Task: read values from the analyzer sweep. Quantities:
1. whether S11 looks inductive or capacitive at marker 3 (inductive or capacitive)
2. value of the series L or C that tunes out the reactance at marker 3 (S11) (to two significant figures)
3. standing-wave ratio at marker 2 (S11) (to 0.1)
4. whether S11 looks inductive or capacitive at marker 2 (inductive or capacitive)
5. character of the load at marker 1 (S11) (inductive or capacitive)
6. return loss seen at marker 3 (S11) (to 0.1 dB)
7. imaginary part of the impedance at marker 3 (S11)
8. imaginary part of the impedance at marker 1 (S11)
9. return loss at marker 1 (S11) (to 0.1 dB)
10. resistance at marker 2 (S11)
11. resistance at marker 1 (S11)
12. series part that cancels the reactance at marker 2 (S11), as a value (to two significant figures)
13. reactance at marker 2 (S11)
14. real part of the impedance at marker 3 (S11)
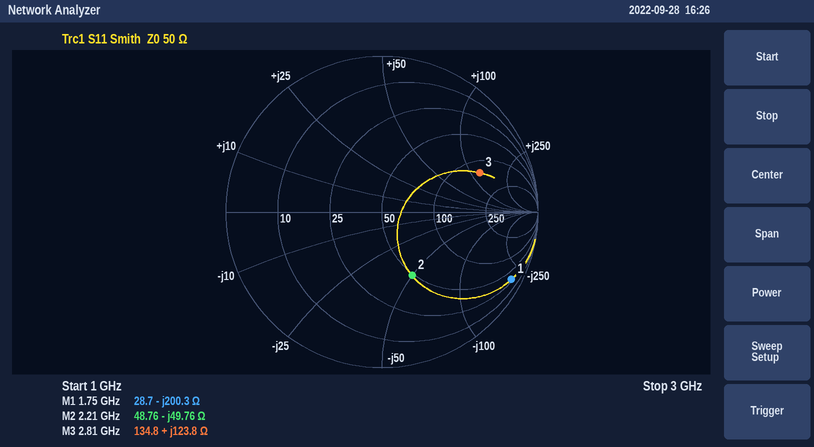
inductive
460 fF
2.6
capacitive
capacitive
3.4 dB
+123.8 Ω
-200.3 Ω
0.6 dB
48.76 Ω
28.7 Ω
3.6 nH
-49.76 Ω
134.8 Ω
